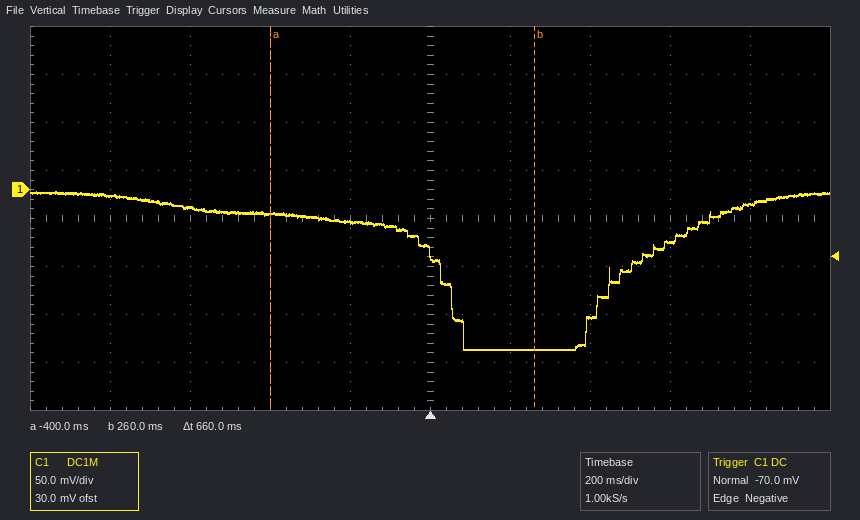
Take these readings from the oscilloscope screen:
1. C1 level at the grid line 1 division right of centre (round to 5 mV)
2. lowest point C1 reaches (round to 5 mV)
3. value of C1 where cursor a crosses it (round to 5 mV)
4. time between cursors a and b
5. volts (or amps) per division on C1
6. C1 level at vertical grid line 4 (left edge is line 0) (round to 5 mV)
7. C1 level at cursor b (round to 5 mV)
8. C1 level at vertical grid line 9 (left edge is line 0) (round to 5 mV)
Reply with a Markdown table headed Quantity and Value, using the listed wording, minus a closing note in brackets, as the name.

| Quantity | Value |
|---|---|
| C1 level at the grid line 1 division right of centre | -165 mV |
| lowest point C1 reaches | -165 mV |
| value of C1 where cursor a crosses it | -25 mV |
| time between cursors a and b | 660 ms |
| volts (or amps) per division on C1 | 50 mV |
| C1 level at vertical grid line 4 (left edge is line 0) | -35 mV |
| C1 level at cursor b | -165 mV |
| C1 level at vertical grid line 9 (left edge is line 0) | -15 mV |
